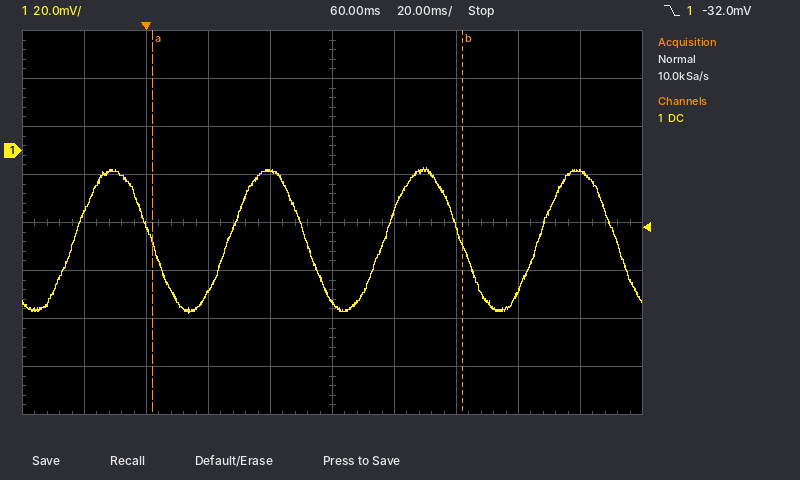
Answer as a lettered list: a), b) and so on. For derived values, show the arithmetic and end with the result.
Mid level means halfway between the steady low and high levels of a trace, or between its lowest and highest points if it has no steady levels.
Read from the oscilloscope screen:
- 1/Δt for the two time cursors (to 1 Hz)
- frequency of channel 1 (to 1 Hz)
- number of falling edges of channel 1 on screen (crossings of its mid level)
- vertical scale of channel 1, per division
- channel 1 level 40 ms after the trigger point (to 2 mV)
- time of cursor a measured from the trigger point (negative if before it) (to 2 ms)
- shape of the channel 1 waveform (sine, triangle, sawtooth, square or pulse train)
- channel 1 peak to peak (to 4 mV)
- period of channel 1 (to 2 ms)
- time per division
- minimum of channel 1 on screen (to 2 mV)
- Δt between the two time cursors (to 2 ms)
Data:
a) 1 / 100 ms ≈ 10 Hz
b) 1 / 50 ms ≈ 20 Hz
c) 4
d) 20 mV
e) -8 mV
f) +2 ms
g) sine
h) 60 mV
i) 50 ms
j) 20 ms
k) -68 mV
l) 100 ms
